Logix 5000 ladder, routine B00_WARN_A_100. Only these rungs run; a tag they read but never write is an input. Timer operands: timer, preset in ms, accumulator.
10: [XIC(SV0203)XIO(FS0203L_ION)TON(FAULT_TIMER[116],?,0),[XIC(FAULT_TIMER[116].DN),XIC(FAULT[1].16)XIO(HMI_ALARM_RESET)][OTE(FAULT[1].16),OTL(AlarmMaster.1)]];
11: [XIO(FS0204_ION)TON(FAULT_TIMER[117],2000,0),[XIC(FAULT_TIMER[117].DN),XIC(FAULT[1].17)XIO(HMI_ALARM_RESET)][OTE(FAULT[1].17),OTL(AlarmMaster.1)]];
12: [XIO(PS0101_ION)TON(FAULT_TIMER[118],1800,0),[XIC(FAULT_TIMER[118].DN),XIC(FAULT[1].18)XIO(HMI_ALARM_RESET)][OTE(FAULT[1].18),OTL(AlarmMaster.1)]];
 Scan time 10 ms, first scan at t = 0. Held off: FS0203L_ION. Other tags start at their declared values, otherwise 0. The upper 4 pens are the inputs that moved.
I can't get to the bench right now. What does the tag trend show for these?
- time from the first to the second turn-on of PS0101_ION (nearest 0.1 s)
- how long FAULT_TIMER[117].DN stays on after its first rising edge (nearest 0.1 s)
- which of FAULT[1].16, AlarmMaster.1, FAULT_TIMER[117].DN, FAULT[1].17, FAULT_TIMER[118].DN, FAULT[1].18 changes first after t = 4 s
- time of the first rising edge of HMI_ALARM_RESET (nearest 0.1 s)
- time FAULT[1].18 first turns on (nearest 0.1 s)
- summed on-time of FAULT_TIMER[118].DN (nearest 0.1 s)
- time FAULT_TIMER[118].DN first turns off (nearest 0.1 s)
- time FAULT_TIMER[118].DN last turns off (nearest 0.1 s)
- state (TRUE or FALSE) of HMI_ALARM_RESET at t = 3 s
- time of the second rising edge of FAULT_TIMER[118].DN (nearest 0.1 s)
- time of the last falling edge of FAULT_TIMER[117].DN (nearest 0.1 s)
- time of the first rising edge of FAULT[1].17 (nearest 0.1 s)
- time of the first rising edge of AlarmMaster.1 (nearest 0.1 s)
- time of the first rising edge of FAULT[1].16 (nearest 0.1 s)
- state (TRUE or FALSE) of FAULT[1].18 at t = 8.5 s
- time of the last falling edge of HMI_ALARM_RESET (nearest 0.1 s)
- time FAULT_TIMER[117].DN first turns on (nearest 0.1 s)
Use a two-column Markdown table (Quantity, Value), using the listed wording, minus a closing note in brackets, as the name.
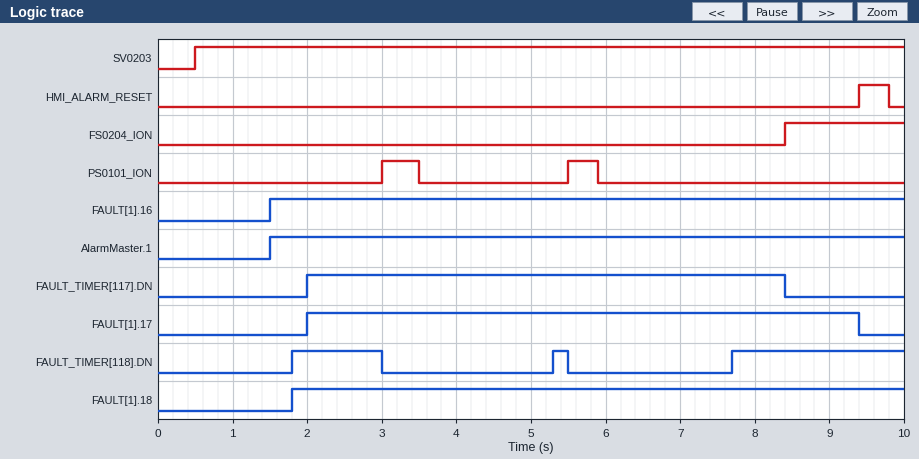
| Quantity | Value |
|---|---|
| time from the first to the second turn-on of PS0101_ION | 2.5 s |
| how long FAULT_TIMER[117].DN stays on after its first rising edge | 6.4 s |
| which of FAULT[1].16, AlarmMaster.1, FAULT_TIMER[117].DN, FAULT[1].17, FAULT_TIMER[118].DN, FAULT[1].18 changes first after t = 4 s | FAULT_TIMER[118].DN |
| time of the first rising edge of HMI_ALARM_RESET | 9.4 s |
| time FAULT[1].18 first turns on | 1.8 s |
| summed on-time of FAULT_TIMER[118].DN | 3.7 s |
| time FAULT_TIMER[118].DN first turns off | 3.0 s |
| time FAULT_TIMER[118].DN last turns off | 5.5 s |
| state (TRUE or FALSE) of HMI_ALARM_RESET at t = 3 s | FALSE |
| time of the second rising edge of FAULT_TIMER[118].DN | 5.3 s |
| time of the last falling edge of FAULT_TIMER[117].DN | 8.4 s |
| time of the first rising edge of FAULT[1].17 | 2.0 s |
| time of the first rising edge of AlarmMaster.1 | 1.5 s |
| time of the first rising edge of FAULT[1].16 | 1.5 s |
| state (TRUE or FALSE) of FAULT[1].18 at t = 8.5 s | TRUE |
| time of the last falling edge of HMI_ALARM_RESET | 9.8 s |
| time FAULT_TIMER[117].DN first turns on | 2.0 s |
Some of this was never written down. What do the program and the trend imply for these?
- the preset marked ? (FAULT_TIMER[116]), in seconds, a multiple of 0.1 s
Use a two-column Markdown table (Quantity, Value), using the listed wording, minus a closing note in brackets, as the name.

| Quantity | Value |
|---|---|
| the preset marked ? (FAULT_TIMER[116]), in seconds, a multiple of 0.1 s | 1.0 s |
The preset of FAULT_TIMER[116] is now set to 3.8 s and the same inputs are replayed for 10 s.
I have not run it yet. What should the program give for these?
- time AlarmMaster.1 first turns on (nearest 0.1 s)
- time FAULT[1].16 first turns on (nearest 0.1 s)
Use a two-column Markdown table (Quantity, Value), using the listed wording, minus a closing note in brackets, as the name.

| Quantity | Value |
|---|---|
| time AlarmMaster.1 first turns on | 1.8 s |
| time FAULT[1].16 first turns on | 4.3 s |
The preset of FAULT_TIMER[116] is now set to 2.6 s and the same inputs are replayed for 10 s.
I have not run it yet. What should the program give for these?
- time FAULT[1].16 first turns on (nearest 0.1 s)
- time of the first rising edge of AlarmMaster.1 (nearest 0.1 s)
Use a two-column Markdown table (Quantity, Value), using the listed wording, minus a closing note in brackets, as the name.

| Quantity | Value |
|---|---|
| time FAULT[1].16 first turns on | 3.1 s |
| time of the first rising edge of AlarmMaster.1 | 1.8 s |
